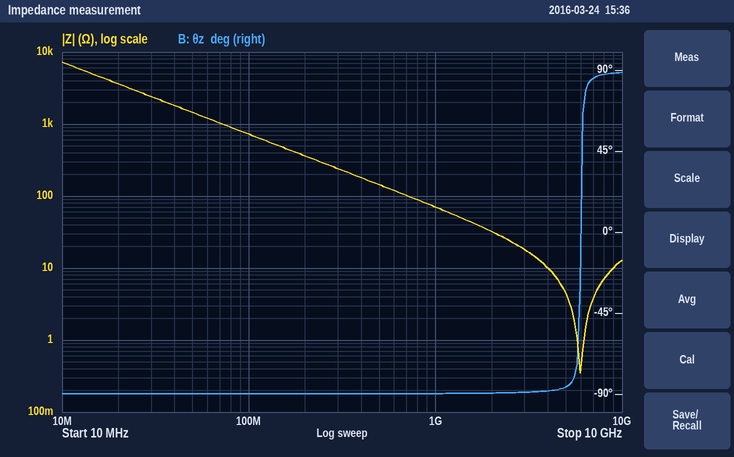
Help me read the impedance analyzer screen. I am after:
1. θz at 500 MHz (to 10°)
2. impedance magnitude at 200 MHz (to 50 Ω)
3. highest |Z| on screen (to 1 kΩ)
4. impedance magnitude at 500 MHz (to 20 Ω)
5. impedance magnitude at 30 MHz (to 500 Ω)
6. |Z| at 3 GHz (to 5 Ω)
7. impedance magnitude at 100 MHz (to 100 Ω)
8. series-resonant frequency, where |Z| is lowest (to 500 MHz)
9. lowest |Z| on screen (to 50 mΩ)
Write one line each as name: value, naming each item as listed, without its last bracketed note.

θz at 500 MHz: -90°
impedance magnitude at 200 MHz: 350 Ω
highest |Z| on screen: 7 kΩ
impedance magnitude at 500 MHz: 140 Ω
impedance magnitude at 30 MHz: 2.5 kΩ
|Z| at 3 GHz: 20 Ω
impedance magnitude at 100 MHz: 700 Ω
series-resonant frequency, where |Z| is lowest: 6.0 GHz
lowest |Z| on screen: 350 mΩ
